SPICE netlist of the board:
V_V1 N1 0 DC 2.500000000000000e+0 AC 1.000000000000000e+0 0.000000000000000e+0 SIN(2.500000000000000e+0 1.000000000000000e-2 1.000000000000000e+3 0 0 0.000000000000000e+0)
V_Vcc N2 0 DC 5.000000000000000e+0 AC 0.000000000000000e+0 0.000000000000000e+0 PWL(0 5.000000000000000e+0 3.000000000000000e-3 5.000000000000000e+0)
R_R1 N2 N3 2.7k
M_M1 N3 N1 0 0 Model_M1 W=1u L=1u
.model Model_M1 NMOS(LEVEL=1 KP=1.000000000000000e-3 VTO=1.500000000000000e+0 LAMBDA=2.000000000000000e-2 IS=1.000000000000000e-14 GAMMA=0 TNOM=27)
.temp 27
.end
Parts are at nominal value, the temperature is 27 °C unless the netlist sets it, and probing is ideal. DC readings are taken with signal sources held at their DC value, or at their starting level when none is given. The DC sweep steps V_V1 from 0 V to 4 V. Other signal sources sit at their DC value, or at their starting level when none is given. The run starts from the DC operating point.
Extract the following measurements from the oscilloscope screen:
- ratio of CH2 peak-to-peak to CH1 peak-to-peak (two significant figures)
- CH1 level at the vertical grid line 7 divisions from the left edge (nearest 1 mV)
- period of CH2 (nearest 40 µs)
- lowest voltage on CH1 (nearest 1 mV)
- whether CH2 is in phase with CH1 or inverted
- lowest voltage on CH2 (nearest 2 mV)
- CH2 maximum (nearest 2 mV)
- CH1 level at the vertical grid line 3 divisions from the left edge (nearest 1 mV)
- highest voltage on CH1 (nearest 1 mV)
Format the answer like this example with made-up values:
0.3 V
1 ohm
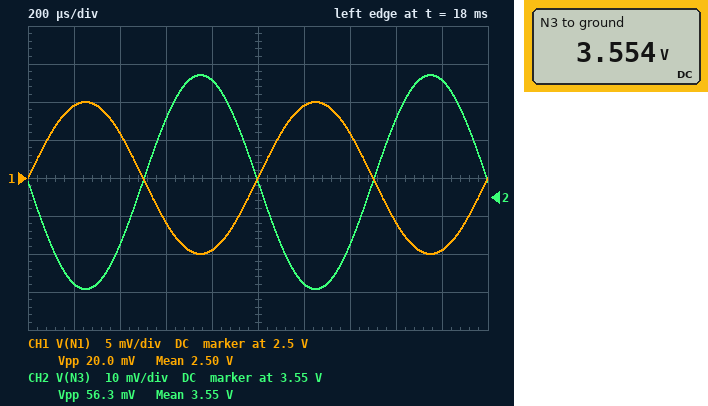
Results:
2.8
2.506 V
1.00 ms
2.490 V
inverted
3.526 V
3.582 V
2.494 V
2.510 V
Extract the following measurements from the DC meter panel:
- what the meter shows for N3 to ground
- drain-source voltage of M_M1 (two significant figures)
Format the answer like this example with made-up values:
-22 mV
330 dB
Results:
3.554 V
3.6 V
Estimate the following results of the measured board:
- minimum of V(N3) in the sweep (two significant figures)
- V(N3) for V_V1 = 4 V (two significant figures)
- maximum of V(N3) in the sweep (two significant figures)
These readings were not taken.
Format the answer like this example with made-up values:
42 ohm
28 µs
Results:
730 mV
730 mV
5.0 V
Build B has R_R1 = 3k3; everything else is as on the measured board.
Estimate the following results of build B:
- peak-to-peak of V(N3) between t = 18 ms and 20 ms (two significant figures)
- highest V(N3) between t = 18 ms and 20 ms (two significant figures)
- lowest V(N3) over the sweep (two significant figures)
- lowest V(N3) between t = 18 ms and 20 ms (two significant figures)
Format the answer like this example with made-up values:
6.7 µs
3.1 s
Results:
68 mV
3.3 V
600 mV
3.2 V
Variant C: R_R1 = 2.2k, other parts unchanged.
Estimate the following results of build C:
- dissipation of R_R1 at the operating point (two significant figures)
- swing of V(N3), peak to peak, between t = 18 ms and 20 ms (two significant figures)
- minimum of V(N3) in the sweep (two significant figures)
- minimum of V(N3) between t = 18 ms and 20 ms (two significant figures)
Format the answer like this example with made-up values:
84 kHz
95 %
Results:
640 µW
46 mV
890 mV
3.8 V
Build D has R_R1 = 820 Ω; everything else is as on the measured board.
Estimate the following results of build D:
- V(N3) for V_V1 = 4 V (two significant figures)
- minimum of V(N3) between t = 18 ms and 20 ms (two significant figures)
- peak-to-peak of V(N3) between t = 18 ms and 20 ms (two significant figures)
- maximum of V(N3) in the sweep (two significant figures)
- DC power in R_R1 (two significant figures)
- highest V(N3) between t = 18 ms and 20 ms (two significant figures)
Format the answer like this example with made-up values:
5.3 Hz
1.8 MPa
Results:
2.3 V
4.5 V
18 mV
5.0 V
240 µW
4.6 V
